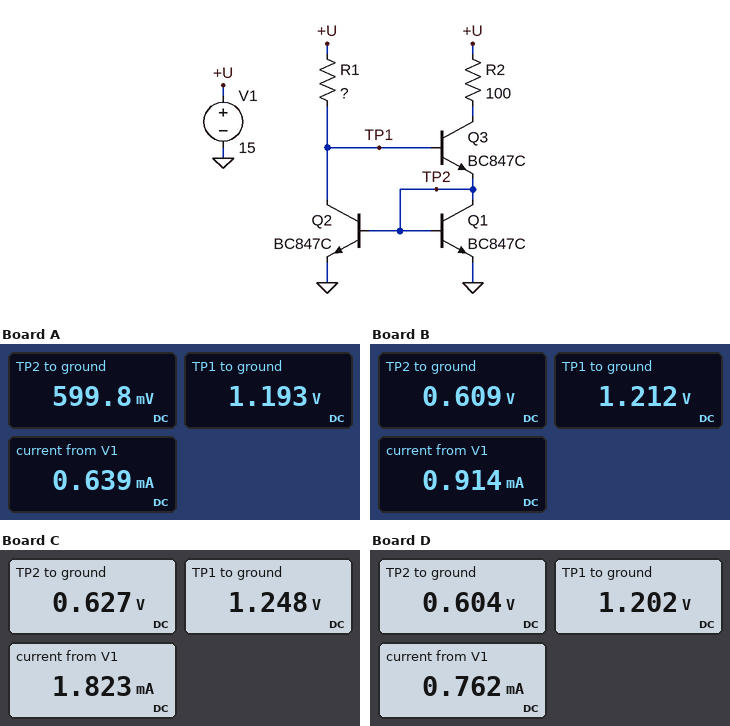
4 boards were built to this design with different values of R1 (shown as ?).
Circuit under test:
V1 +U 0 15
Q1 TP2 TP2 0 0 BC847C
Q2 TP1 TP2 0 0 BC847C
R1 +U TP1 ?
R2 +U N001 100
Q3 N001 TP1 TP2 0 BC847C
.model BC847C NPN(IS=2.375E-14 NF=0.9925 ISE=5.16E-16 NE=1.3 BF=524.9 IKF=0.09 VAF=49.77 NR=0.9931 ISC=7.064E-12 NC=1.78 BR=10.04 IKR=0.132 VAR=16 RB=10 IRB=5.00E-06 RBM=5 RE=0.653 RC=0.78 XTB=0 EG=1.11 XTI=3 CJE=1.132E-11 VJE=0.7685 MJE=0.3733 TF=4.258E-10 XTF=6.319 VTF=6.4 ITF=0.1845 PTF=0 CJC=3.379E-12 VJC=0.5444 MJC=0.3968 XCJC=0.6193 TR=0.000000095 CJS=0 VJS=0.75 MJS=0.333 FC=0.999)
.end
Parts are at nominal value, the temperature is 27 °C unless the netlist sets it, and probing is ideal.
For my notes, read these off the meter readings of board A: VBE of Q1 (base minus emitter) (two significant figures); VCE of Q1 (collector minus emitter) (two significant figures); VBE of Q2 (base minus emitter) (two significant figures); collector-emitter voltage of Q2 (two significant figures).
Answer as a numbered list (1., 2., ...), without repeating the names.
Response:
1. 600 mV
2. 600 mV
3. 600 mV
4. 1.2 V
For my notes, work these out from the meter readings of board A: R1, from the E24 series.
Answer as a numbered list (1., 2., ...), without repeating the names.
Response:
1. 43 kΩ
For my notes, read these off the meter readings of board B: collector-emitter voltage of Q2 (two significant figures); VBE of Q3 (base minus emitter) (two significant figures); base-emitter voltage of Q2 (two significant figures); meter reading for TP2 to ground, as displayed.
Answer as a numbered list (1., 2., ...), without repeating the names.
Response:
1. 1.2 V
2. 600 mV
3. 610 mV
4. 0.609 V
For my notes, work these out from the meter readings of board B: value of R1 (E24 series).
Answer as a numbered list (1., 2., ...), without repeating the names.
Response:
1. 30 kΩ
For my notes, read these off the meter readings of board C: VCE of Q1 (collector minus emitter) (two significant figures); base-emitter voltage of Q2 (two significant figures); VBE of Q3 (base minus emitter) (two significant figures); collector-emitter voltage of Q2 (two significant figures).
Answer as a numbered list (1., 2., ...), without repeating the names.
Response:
1. 630 mV
2. 630 mV
3. 620 mV
4. 1.2 V
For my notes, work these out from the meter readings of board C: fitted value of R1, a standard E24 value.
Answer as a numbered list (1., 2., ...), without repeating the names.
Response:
1. 15 kΩ
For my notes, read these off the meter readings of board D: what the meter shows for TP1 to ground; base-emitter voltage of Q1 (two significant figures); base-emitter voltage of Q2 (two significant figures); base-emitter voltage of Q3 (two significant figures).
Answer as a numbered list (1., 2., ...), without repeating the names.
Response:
1. 1.202 V
2. 600 mV
3. 600 mV
4. 600 mV
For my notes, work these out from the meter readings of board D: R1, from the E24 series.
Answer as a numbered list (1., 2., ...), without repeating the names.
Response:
1. 36 kΩ
